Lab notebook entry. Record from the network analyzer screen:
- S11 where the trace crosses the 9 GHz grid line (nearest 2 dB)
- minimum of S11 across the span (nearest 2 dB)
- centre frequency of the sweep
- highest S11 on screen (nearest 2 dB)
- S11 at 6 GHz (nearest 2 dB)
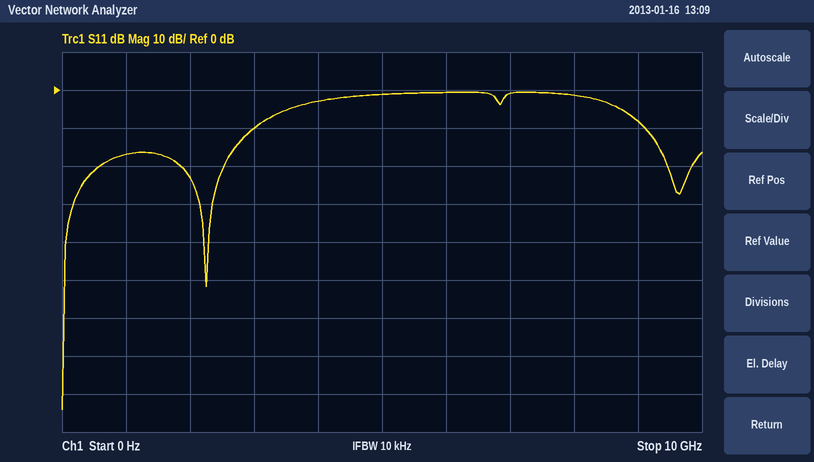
-8 dB
-84 dB
5 GHz
0 dB
0 dB
